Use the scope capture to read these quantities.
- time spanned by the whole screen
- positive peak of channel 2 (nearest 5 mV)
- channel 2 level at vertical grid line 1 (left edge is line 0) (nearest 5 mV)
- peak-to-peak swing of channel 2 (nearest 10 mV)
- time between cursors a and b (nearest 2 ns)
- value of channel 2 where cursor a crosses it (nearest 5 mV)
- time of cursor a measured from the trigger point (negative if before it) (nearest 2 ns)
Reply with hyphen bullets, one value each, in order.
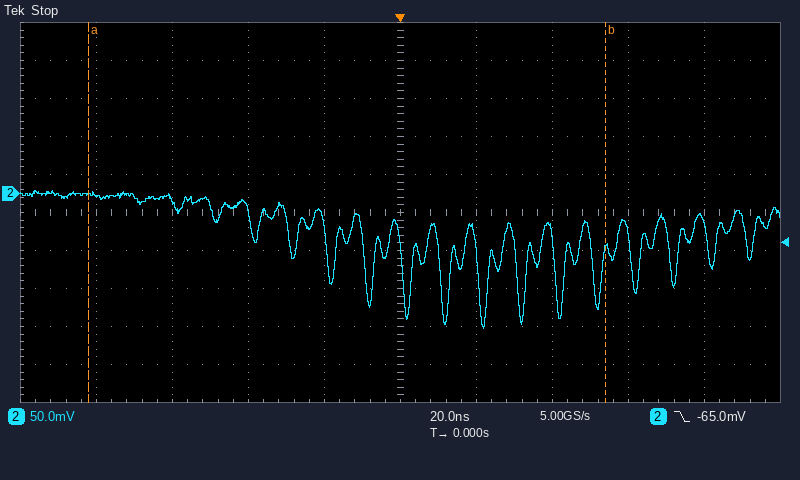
- 200 ns
- 5 mV
- 0 mV
- 180 mV
- 136 ns
- 0 mV
- -82 ns
